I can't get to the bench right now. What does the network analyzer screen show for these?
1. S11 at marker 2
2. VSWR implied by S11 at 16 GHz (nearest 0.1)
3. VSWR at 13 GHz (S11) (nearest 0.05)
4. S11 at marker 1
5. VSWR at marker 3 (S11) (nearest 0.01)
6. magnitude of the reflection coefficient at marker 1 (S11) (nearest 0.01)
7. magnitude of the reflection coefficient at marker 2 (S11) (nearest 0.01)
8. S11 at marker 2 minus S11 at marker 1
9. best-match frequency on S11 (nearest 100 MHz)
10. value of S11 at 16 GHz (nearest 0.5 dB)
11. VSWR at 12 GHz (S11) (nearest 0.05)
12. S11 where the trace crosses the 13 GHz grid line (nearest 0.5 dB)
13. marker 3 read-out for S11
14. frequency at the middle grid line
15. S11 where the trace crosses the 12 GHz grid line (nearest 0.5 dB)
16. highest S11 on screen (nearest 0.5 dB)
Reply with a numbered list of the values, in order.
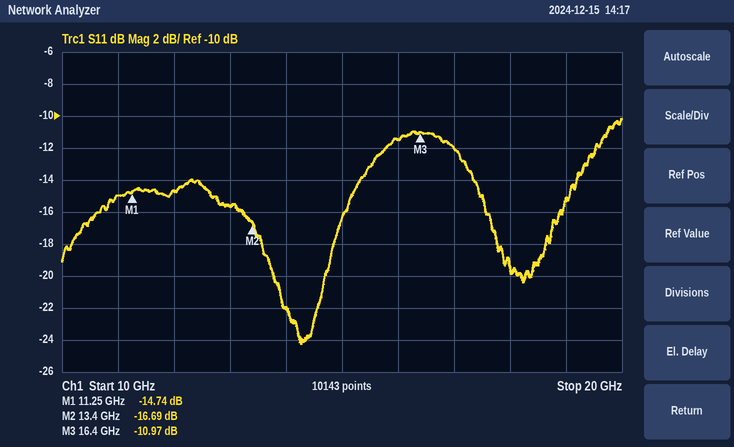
1. -16.69 dB
2. 1.7
3. 1.40
4. -14.74 dB
5. 1.79
6. 0.18
7. 0.15
8. -1.95 dB
9. 14.3 GHz
10. -11.5 dB
11. 1.45
12. -15.5 dB
13. -10.97 dB
14. 15 GHz
15. -14.5 dB
16. -10.0 dB
